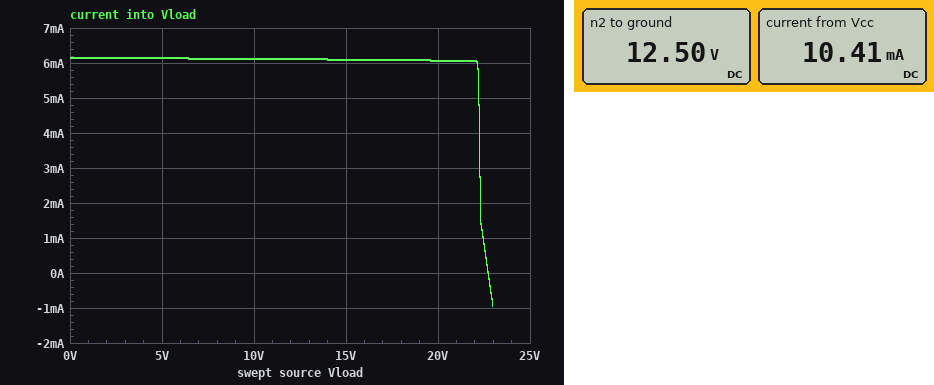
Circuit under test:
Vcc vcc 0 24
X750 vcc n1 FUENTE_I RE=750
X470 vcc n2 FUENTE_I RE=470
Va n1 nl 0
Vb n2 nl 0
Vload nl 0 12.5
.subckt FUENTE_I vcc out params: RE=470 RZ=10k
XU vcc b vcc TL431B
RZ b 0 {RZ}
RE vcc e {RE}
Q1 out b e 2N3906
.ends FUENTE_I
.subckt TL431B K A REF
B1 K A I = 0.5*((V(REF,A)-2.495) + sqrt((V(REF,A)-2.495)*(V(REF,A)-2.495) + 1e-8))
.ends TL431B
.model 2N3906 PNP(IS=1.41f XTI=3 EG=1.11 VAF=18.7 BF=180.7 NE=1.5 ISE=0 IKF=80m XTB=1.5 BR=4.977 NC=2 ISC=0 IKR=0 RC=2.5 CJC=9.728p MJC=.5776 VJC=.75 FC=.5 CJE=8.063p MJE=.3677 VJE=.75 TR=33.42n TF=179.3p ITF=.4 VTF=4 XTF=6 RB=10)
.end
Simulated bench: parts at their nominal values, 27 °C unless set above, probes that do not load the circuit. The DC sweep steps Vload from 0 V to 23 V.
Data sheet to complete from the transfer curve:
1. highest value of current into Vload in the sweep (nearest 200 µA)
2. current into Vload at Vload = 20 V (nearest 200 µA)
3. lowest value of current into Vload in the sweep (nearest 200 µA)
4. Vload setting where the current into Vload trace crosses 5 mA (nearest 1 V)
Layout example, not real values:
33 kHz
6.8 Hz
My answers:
6.2 mA
6.0 mA
-1.0 mA
22 V
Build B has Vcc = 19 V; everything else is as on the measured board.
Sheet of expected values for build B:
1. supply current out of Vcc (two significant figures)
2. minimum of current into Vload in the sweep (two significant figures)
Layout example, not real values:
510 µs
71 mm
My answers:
9.4 mA
-18 mA
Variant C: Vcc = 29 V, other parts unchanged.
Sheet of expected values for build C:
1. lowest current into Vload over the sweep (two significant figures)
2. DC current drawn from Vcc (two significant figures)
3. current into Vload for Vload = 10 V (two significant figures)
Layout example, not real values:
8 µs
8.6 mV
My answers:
6.1 mA
11 mA
6.1 mA
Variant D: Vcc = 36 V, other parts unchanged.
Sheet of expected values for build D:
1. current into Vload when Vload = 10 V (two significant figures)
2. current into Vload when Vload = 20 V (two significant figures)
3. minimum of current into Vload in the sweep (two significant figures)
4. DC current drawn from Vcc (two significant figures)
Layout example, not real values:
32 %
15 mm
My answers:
6.2 mA
6.1 mA
6.1 mA
13 mA
